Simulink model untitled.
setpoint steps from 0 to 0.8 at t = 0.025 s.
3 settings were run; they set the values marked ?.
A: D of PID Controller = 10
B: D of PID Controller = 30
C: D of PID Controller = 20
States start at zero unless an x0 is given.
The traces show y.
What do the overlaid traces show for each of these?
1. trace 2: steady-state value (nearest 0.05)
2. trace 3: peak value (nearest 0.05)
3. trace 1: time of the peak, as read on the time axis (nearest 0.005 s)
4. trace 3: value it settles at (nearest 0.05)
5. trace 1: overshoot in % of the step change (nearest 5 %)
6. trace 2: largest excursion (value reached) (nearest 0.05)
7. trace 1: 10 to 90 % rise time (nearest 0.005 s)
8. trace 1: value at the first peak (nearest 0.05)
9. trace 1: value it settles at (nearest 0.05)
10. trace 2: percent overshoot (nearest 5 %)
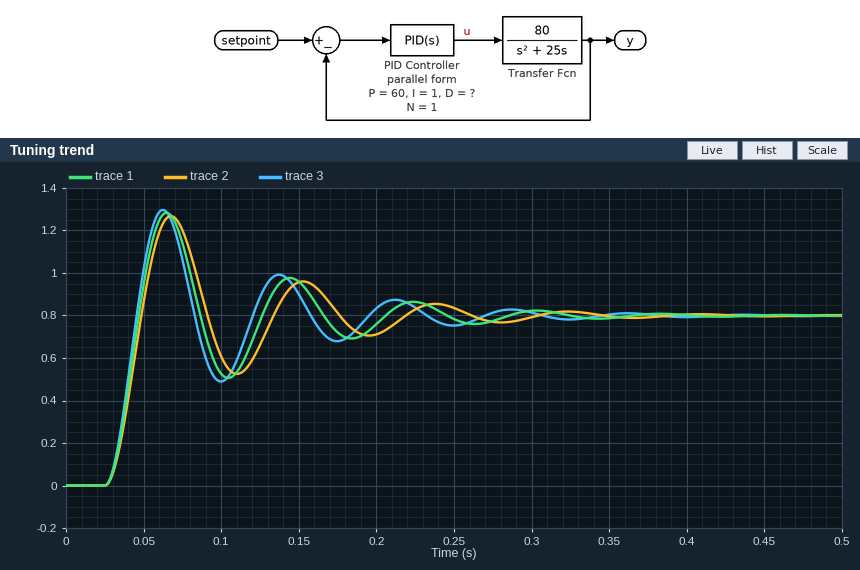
0.80
1.30
0.065 s
0.80
60 %
1.25
0.015 s
1.30
0.80
60 %
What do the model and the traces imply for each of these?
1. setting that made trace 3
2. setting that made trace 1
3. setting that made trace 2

B
C
A
